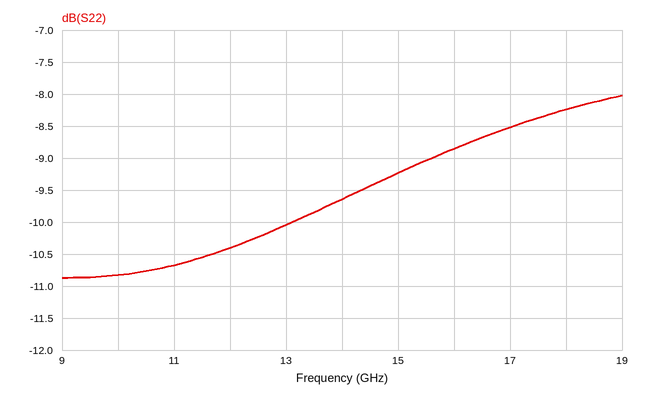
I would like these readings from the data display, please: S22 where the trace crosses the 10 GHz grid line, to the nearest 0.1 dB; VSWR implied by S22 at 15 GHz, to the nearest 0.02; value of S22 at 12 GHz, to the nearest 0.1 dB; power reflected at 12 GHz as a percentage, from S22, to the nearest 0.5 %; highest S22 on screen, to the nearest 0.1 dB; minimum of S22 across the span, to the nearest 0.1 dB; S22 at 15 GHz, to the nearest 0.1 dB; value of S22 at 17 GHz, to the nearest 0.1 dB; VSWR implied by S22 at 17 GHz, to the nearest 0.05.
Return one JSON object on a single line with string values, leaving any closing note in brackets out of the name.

{"S22 where the trace crosses the 10 GHz grid line, to the nearest 0.1 dB": "-10.8 dB", "VSWR implied by S22 at 15 GHz, to the nearest 0.02": "2.06", "value of S22 at 12 GHz, to the nearest 0.1 dB": "-10.4 dB", "power reflected at 12 GHz as a percentage, from S22, to the nearest 0.5 %": "9.0 %", "highest S22 on screen, to the nearest 0.1 dB": "-8.0 dB", "minimum of S22 across the span, to the nearest 0.1 dB": "-10.9 dB", "S22 at 15 GHz, to the nearest 0.1 dB": "-9.2 dB", "value of S22 at 17 GHz, to the nearest 0.1 dB": "-8.5 dB", "VSWR implied by S22 at 17 GHz, to the nearest 0.05": "2.20"}
